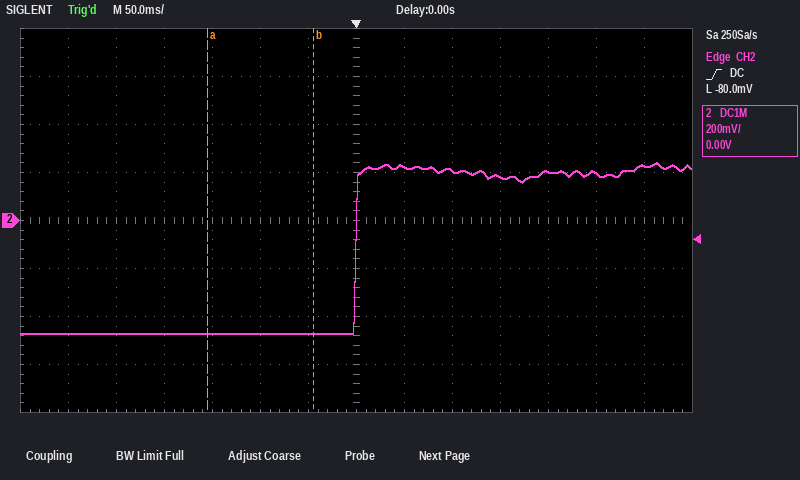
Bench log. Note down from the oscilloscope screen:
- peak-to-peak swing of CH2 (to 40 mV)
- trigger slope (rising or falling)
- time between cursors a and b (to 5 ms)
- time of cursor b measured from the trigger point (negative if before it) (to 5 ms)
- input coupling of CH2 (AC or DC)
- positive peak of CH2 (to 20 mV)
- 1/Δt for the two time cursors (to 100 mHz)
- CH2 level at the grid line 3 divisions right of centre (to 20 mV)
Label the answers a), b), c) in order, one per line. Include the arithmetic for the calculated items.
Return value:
a) 720 mV
b) rising
c) 110 ms
d) -45 ms
e) DC
f) 240 mV
g) 1 / 110 ms ≈ 9.1 Hz
h) 180 mV
